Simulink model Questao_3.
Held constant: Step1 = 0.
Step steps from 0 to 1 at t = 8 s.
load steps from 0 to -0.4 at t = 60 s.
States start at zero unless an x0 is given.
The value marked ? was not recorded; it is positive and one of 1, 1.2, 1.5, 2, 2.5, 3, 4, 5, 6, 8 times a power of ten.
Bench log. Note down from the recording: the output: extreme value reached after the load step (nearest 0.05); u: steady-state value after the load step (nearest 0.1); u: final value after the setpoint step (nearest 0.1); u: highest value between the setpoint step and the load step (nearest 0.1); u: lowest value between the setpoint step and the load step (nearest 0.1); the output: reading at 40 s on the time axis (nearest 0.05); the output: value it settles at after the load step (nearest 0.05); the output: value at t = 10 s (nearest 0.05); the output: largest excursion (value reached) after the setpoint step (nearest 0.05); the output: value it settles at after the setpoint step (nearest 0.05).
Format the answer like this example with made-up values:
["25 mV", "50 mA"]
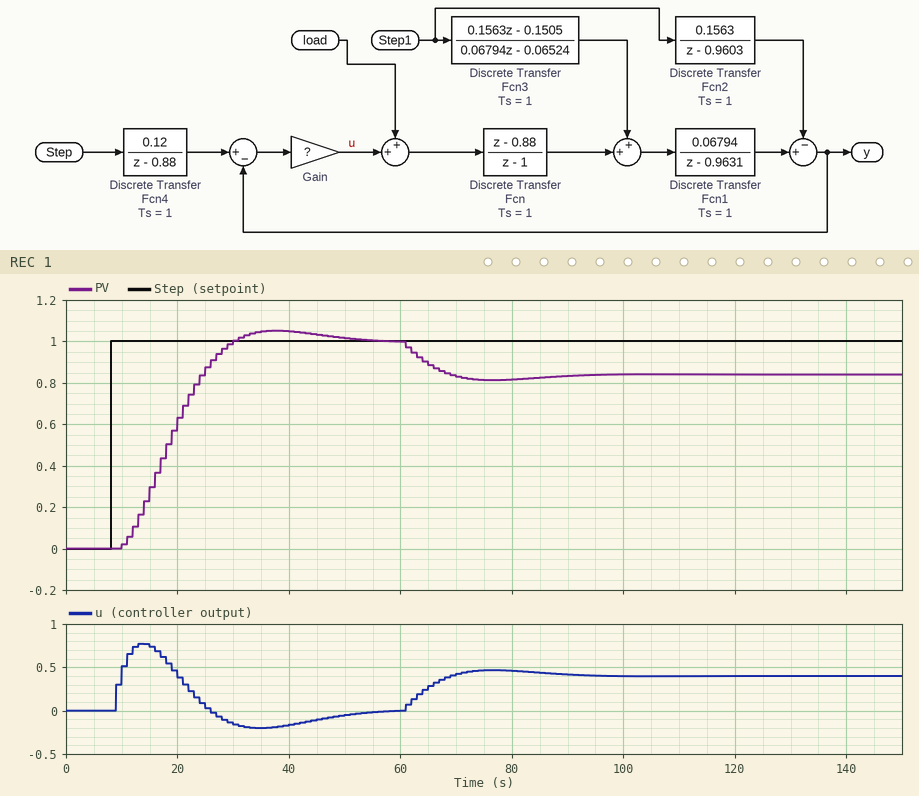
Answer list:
["0.80", "0.4", "0.0", "0.8", "-0.2", "1.05", "0.85", "0.00", "1.05", "1.00"]
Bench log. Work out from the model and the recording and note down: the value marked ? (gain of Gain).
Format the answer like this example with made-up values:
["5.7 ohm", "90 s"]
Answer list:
["2.5"]
